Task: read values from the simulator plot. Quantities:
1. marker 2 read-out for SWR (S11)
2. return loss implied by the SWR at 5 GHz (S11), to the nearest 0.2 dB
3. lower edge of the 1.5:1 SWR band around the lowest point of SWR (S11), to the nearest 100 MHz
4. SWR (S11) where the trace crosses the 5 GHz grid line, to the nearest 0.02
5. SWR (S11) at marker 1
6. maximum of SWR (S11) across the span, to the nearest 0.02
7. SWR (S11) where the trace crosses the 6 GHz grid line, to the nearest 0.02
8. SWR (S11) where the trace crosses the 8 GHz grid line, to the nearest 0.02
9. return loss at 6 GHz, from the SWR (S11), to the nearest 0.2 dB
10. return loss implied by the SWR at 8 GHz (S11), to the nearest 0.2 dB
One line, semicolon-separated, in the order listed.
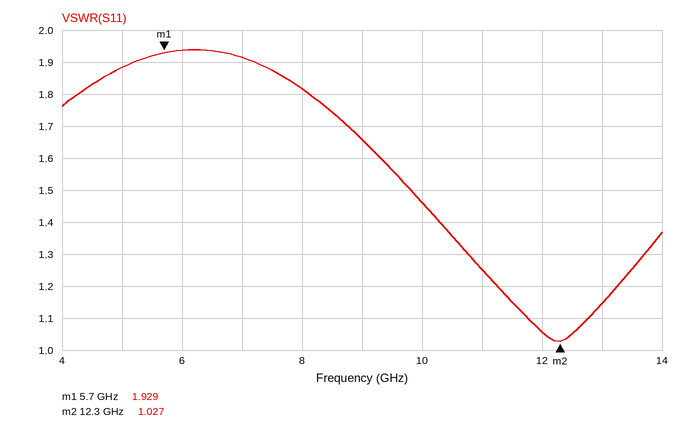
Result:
1.027; 10.2 dB; 9.8 GHz; 1.88; 1.929; 1.94; 1.94; 1.82; 10.0 dB; 10.8 dB
